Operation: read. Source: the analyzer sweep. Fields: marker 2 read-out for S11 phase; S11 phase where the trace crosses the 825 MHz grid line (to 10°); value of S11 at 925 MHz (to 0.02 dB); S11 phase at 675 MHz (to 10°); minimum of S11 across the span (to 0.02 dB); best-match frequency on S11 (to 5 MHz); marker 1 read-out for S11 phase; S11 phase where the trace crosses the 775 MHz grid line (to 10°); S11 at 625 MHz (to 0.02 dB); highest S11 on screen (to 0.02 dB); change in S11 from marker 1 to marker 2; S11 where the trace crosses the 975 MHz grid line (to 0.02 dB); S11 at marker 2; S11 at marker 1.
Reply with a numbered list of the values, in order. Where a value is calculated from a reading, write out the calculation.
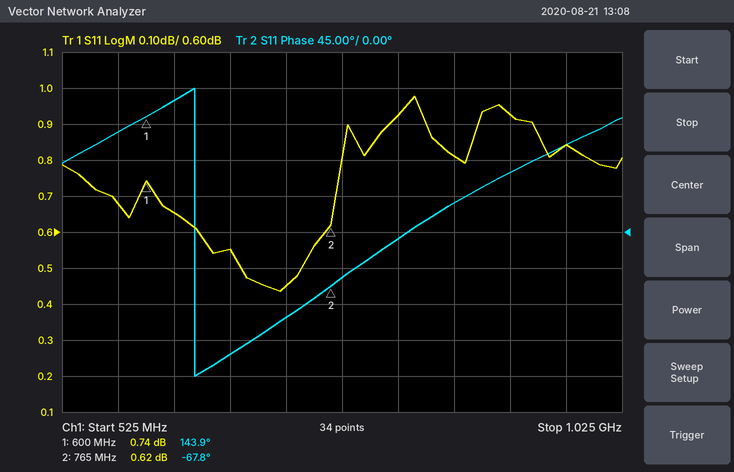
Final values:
1. -67.8°
2. -10°
3. 0.92 dB
4. -150°
5. 0.44 dB
6. 720 MHz
7. 143.9°
8. -60°
9. 0.66 dB
10. 0.98 dB
11. 0.62 − (0.74) = -0.12 dB
12. 0.84 dB
13. 0.62 dB
14. 0.74 dB
